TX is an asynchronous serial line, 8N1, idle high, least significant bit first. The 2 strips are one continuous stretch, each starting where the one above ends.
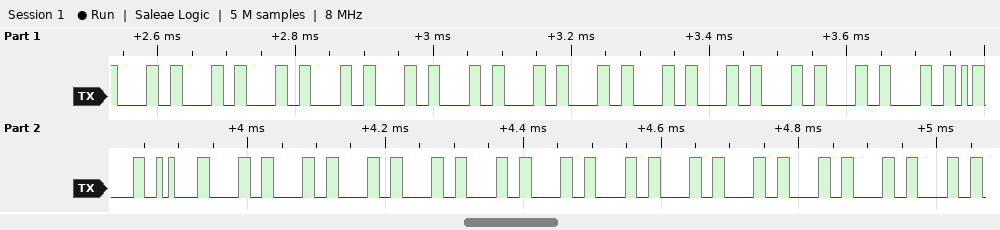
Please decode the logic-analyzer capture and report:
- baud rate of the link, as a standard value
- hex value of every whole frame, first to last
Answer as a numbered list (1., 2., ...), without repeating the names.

1. 115200 baud
2. 30 30 30 30 30 30 30 30 30 30 30 30 30 0D 0A 30 30 30 30 30 30 30 30 30 30 30 30
